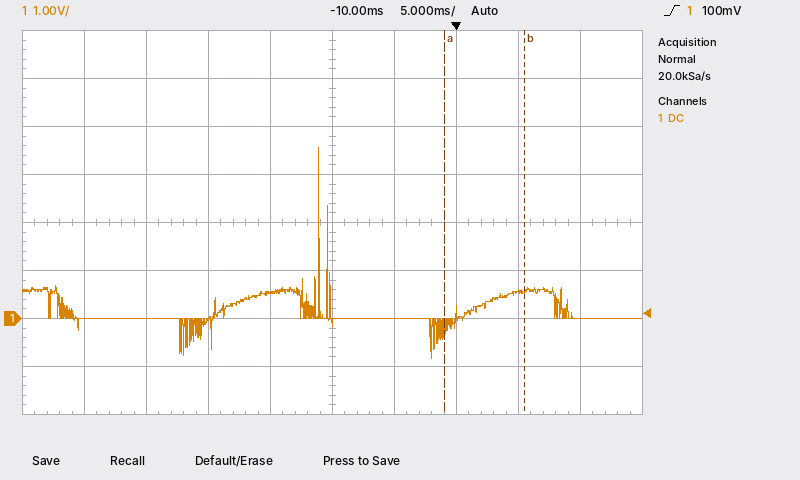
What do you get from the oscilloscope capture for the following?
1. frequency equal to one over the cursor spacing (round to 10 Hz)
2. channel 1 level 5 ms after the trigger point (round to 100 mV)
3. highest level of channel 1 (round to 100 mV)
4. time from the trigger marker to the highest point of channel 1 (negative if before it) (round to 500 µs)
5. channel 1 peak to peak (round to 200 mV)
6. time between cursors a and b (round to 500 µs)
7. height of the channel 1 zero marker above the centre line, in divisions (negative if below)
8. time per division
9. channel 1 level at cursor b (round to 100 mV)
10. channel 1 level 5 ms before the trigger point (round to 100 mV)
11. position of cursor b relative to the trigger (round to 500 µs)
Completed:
150 Hz
600 mV
3.6 V
-11.0 ms
4.4 V
6.5 ms
-2.0 div
5 ms
600 mV
0.0 V
+5.5 ms
